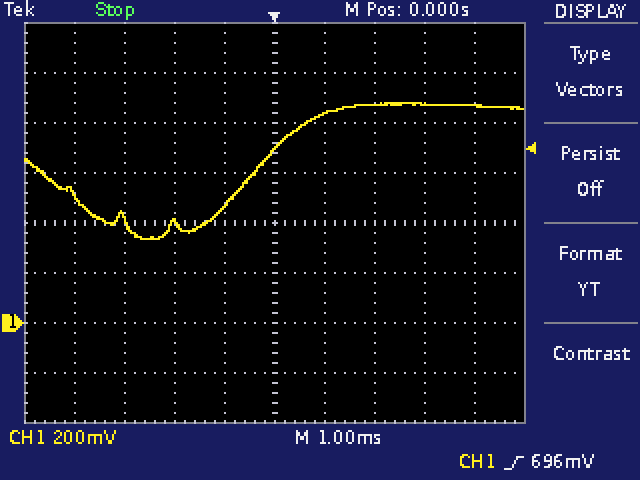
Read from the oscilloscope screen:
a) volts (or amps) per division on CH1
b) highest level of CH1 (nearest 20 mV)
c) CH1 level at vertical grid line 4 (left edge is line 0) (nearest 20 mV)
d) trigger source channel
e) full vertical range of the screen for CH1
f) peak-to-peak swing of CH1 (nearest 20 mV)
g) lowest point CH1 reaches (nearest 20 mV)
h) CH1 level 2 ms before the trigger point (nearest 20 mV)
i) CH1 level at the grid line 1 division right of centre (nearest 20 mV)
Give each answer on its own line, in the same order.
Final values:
200 mV
880 mV
460 mV
CH1
1.6 V
540 mV
340 mV
400 mV
840 mV
